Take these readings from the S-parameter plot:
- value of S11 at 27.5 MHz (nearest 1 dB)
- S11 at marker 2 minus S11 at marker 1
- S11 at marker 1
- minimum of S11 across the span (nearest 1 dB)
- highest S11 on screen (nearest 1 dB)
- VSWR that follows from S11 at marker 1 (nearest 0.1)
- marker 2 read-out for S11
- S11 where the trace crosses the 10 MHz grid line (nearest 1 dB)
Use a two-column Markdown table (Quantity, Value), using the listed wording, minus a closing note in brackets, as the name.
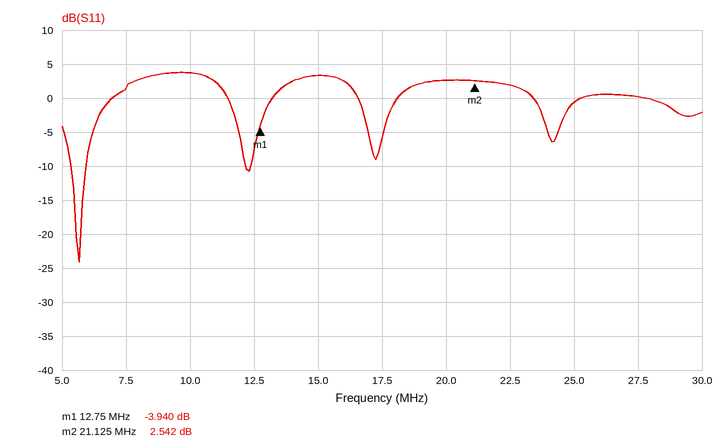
| Quantity | Value |
|---|---|
| value of S11 at 27.5 MHz | 0 dB |
| S11 at marker 2 minus S11 at marker 1 | 6.482 dB |
| S11 at marker 1 | -3.940 dB |
| minimum of S11 across the span | -24 dB |
| highest S11 on screen | 4 dB |
| VSWR that follows from S11 at marker 1 | 4.5 |
| marker 2 read-out for S11 | 2.542 dB |
| S11 where the trace crosses the 10 MHz grid line | 4 dB |
